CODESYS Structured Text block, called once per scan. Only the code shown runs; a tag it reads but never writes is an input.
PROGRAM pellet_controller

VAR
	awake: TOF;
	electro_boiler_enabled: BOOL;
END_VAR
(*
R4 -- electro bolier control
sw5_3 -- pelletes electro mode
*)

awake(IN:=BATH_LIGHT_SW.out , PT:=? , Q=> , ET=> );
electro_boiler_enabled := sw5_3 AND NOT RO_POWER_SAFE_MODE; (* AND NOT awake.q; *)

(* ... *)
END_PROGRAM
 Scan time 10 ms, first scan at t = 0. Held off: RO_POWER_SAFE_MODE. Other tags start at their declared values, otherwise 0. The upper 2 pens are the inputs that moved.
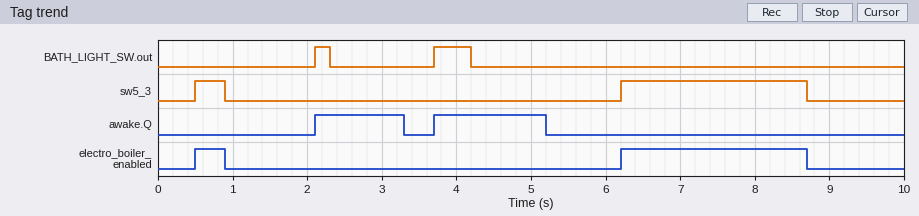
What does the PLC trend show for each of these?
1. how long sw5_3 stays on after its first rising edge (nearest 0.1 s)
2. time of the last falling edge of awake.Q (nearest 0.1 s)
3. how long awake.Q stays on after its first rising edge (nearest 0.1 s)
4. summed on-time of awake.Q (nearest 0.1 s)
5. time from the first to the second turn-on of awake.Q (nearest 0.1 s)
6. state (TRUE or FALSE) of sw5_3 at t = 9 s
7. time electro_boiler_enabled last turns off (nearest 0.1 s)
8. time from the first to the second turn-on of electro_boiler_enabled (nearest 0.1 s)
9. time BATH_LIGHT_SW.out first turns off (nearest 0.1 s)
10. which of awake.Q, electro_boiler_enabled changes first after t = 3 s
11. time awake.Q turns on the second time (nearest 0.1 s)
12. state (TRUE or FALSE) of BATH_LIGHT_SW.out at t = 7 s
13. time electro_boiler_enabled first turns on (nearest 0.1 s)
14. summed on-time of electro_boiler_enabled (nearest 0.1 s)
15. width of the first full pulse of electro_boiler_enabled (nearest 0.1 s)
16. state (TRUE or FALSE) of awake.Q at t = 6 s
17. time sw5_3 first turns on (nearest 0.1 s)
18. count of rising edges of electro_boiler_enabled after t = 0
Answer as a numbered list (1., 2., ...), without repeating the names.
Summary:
1. 0.4 s
2. 5.2 s
3. 1.2 s
4. 2.7 s
5. 1.6 s
6. FALSE
7. 8.7 s
8. 5.7 s
9. 2.3 s
10. awake.Q
11. 3.7 s
12. FALSE
13. 0.5 s
14. 2.9 s
15. 0.4 s
16. FALSE
17. 0.5 s
18. 2
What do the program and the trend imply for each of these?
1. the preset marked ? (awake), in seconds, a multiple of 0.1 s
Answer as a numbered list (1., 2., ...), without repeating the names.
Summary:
1. 1.0 s
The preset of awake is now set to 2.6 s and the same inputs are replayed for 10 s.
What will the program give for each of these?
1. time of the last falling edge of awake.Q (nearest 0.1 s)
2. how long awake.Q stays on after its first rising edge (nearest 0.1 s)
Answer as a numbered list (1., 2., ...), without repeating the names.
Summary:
1. 6.8 s
2. 4.7 s
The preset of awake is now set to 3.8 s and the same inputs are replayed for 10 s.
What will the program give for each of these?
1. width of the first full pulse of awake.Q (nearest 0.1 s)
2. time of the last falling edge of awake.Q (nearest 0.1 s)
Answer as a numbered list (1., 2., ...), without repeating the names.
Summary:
1. 5.9 s
2. 8.0 s
